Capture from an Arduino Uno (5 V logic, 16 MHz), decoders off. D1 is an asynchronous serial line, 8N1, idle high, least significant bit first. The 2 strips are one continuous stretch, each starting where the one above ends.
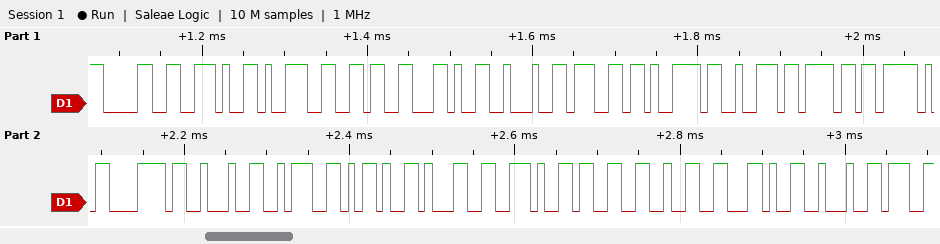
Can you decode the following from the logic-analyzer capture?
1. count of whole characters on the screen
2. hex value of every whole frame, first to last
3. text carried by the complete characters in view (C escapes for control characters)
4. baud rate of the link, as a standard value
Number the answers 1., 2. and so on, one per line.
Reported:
1. 21
2. 30 2E 39 36 2C 22 67 79 72 6F 5F 78 22 3A 2D 31 2E 33 32 2C 22
3. "0.96,\"gyro_x\":-1.32,\""
4. 115200 baud
